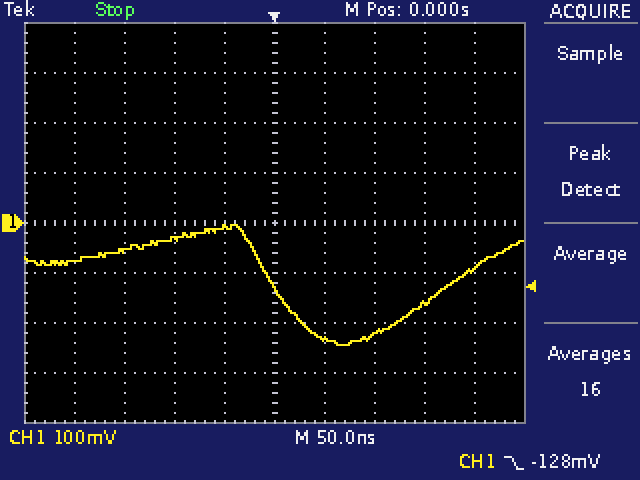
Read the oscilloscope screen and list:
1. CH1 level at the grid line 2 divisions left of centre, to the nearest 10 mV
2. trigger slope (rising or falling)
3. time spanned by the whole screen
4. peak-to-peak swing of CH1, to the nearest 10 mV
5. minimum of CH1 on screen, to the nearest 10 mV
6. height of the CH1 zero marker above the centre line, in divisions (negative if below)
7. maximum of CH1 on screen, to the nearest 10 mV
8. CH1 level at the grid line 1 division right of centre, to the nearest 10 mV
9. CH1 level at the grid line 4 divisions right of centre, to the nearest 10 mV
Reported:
-30 mV
falling
500 ns
240 mV
-240 mV
0.0 div
0 mV
-230 mV
-90 mV
